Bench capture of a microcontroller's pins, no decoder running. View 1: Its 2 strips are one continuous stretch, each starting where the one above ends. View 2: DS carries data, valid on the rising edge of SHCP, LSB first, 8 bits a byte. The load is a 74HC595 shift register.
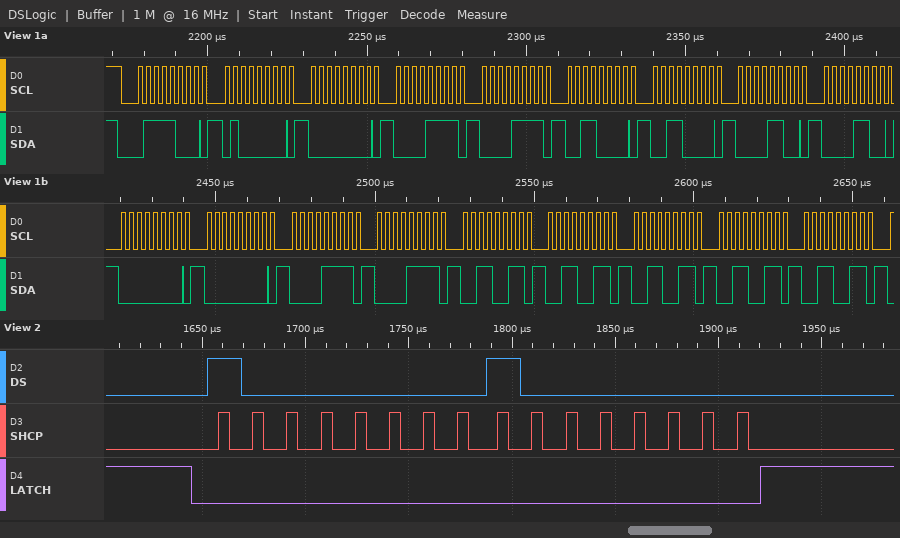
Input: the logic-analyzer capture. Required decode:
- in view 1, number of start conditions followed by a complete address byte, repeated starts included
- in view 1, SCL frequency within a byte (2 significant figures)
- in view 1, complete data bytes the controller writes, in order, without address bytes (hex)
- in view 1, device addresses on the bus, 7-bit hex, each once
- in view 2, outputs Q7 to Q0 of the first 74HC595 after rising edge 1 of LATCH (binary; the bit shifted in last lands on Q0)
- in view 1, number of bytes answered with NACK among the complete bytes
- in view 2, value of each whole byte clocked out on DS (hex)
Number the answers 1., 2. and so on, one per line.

1. 1
2. 400 kHz
3. 40 00 0F 0F 30 30 0C 0C 00 00 0F 0F 33 33 33 33 33
4. 0x3C
5. 10000000
6. 0
7. 0x01 0x01
